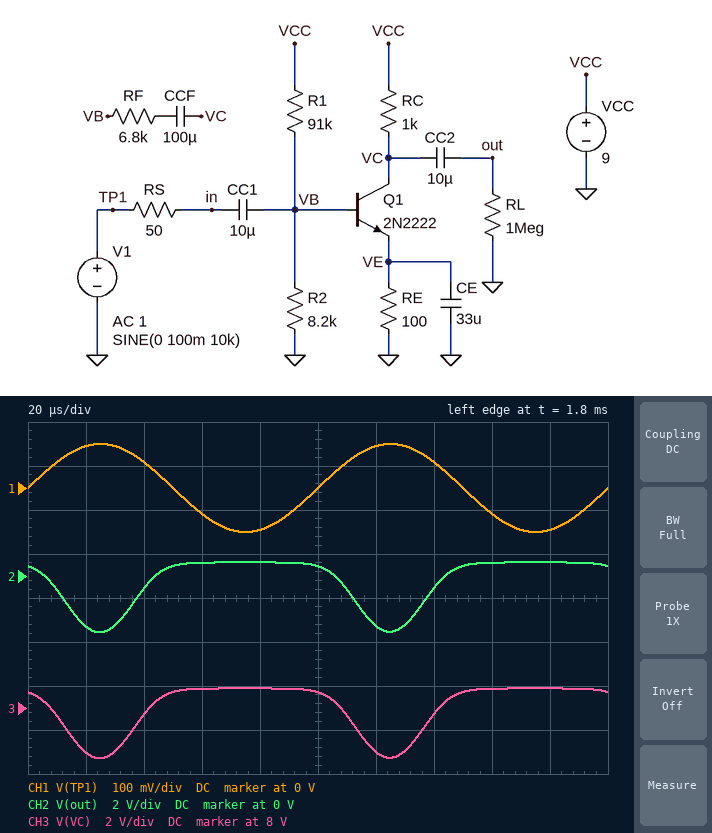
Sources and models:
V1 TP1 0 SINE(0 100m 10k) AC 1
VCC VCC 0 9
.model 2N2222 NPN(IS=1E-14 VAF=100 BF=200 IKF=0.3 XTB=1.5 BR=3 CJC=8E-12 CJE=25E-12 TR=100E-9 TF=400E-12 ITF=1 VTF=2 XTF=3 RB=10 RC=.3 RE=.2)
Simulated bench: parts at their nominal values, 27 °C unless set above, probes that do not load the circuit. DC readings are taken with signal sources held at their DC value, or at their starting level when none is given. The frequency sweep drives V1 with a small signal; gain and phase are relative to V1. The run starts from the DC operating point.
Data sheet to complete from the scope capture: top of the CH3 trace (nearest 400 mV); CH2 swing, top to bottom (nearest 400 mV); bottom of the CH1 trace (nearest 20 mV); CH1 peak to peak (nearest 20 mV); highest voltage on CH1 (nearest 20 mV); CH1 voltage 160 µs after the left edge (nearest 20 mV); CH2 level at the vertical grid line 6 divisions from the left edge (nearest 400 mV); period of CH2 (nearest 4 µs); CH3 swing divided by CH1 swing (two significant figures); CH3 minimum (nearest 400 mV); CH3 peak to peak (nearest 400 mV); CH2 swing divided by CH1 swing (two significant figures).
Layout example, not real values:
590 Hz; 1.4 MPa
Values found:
8.8 V; 3.2 V; -100 mV; 200 mV; 100 mV; -60 mV; -2.4 V; 100 µs; 16; 5.6 V; 3.2 V; 16
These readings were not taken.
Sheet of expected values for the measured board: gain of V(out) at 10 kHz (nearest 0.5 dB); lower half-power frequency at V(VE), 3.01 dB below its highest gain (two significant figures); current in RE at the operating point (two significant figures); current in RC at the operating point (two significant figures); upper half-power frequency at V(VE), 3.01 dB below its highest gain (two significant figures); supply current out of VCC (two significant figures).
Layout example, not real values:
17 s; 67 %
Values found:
26.0 dB; 13 Hz; 730 µA; 730 µA; 230 Hz; 820 µA
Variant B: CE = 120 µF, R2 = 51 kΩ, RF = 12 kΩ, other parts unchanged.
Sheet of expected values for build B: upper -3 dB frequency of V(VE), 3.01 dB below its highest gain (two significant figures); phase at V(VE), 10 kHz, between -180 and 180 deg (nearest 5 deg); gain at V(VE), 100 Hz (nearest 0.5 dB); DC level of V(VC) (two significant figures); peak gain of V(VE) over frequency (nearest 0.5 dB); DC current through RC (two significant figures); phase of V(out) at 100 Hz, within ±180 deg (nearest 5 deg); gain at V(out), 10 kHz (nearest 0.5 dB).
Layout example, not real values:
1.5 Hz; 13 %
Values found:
280 Hz; -90 deg; -15.0 dB; 960 mV; -14.5 dB; 8.0 mA; -110 deg; 28.0 dB
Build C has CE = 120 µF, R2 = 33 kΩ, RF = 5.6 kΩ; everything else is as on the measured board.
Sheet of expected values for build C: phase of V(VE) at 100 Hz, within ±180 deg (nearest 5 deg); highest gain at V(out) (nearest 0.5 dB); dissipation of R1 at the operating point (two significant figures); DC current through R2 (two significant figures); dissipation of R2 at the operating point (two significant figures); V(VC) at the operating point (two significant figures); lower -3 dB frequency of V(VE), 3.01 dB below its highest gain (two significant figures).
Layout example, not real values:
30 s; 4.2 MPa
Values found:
-10 deg; 37.0 dB; 620 µW; 44 µA; 65 µW; 1.5 V; 9.1 Hz
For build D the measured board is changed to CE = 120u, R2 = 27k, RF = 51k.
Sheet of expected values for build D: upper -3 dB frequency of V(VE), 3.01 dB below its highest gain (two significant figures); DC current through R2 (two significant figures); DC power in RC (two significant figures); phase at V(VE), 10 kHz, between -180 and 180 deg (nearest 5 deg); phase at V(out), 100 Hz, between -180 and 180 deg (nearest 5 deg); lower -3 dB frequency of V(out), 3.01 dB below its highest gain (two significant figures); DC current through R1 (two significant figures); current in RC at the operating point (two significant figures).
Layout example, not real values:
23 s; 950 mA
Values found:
320 Hz; 51 µA; 43 mW; -90 deg; -115 deg; 310 Hz; 84 µA; 6.6 mA
